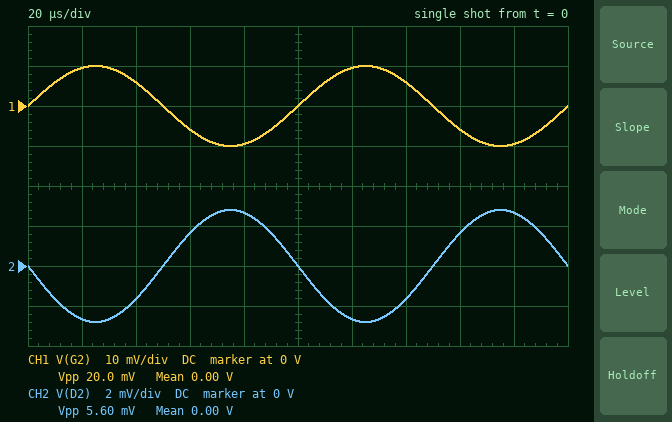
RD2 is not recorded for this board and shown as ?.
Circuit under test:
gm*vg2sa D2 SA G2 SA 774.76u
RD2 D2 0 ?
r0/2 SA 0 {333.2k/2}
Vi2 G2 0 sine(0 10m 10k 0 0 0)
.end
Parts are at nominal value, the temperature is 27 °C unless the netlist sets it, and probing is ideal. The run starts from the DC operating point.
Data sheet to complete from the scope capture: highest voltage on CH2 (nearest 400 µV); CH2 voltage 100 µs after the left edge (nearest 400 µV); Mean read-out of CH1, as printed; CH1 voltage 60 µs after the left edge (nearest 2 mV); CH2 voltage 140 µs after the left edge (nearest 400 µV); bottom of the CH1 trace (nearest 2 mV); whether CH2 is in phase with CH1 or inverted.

2.8 mV
0 V
0.00 V
-6 mV
-1.6 mV
-10 mV
inverted
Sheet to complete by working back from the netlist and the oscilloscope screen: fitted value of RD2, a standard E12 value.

47 kΩ
